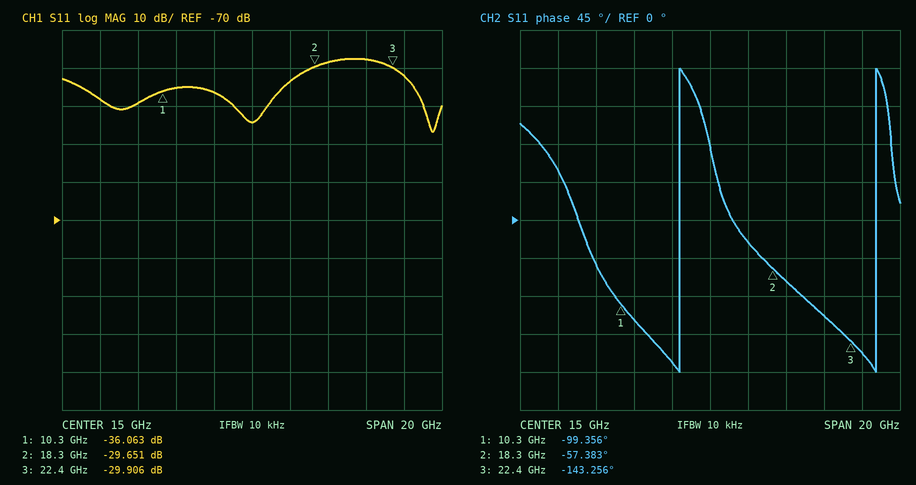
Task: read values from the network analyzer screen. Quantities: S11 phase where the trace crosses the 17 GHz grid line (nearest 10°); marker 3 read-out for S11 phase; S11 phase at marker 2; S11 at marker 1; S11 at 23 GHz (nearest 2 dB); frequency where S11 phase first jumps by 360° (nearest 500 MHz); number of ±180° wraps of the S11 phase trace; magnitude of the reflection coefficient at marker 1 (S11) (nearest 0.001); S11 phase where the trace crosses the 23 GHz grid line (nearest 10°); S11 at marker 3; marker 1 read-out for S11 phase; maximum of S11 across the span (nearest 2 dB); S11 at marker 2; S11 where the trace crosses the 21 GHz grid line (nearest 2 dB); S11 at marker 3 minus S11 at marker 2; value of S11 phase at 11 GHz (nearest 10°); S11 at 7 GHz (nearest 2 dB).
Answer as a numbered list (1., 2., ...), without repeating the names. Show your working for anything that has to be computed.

1. -30°
2. -143.256°
3. -57.383°
4. -36.063 dB
5. -32 dB
6. 13.5 GHz
7. 2
8. 10^(-36.063/20) ≈ 0.016
9. -160°
10. -29.906 dB
11. -99.356°
12. -28 dB
13. -29.651 dB
14. -28 dB
15. -29.906 − (-29.651) = -0.255 dB
16. -120°
17. -38 dB
